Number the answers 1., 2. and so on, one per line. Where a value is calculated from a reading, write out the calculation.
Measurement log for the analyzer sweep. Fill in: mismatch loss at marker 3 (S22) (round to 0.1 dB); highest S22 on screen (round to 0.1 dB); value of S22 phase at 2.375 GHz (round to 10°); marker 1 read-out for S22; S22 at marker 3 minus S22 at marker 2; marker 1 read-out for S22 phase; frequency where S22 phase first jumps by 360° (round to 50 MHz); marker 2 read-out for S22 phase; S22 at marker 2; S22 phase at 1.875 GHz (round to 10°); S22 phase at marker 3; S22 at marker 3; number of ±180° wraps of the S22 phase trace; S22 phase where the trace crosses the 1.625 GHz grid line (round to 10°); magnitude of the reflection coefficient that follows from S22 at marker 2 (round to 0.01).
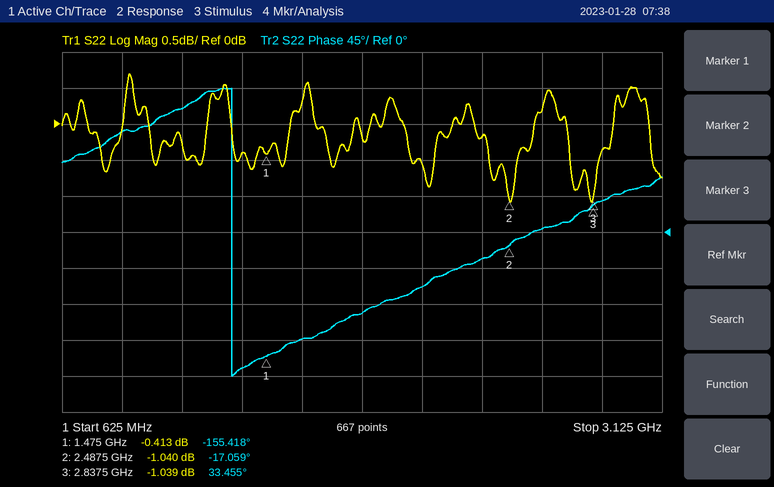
1. −10 log10(1 − 10^(-1.039/10)) ≈ 6.7 dB
2. 0.7 dB
3. -30°
4. -0.413 dB
5. -1.039 − (-1.04) = 0.001 dB
6. -155.418°
7. 1.35 GHz
8. -17.059°
9. -1.040 dB
10. -100°
11. 33.455°
12. -1.039 dB
13. 1
14. -130°
15. 10^(-1.04/20) ≈ 0.89
